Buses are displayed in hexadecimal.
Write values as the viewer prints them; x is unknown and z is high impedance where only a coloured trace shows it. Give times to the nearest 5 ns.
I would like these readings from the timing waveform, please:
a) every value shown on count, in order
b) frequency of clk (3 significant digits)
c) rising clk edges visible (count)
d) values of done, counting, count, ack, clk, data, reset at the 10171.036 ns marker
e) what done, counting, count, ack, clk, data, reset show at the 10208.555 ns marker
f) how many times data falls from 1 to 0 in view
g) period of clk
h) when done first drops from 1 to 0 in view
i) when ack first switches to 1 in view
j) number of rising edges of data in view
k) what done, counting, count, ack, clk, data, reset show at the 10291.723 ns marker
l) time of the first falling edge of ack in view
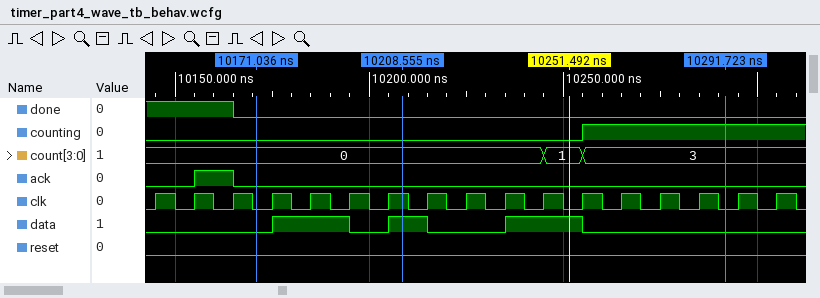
0, 1, 3
100 MHz
17
done=0, counting=0, count=0, ack=0, clk=0, data=0, reset=0
done=0, counting=0, count=0, ack=0, clk=1, data=1, reset=0
3
10 ns
10165 ns
10155 ns
3
done=0, counting=1, count=3, ack=0, clk=0, data=0, reset=0
10165 ns
